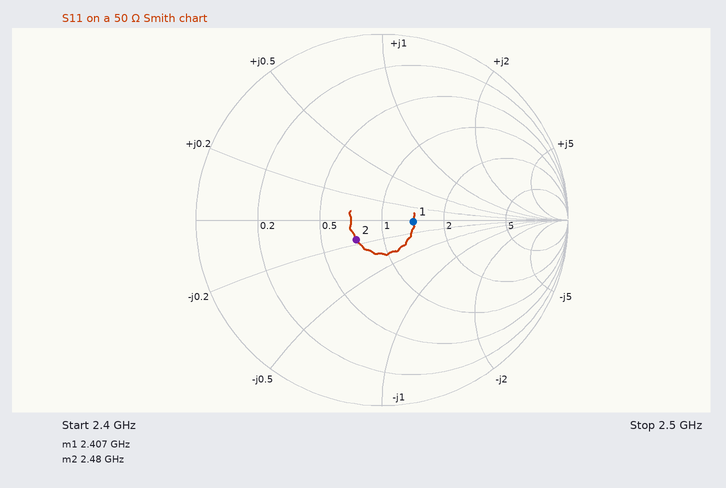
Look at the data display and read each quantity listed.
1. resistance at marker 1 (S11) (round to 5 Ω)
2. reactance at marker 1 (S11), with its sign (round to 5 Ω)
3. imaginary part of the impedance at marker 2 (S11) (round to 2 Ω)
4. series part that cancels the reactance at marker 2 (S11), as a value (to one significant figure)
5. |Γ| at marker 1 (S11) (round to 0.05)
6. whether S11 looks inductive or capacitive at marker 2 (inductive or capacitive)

70 Ω
0 Ω
-8 Ω
500 pH
0.15
capacitive
